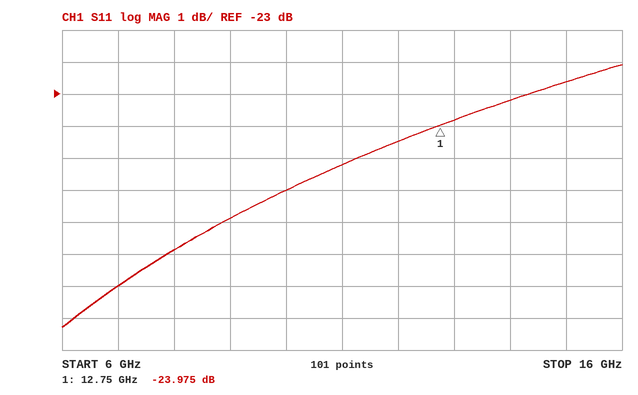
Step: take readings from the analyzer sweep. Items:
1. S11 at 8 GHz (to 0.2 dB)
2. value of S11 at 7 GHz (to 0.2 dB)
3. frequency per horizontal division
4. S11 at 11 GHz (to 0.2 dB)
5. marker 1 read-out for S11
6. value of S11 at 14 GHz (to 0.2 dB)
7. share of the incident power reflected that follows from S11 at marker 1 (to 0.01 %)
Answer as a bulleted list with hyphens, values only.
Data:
- -27.8 dB
- -29.0 dB
- 1 GHz
- -25.2 dB
- -23.975 dB
- -23.2 dB
- 0.40 %
